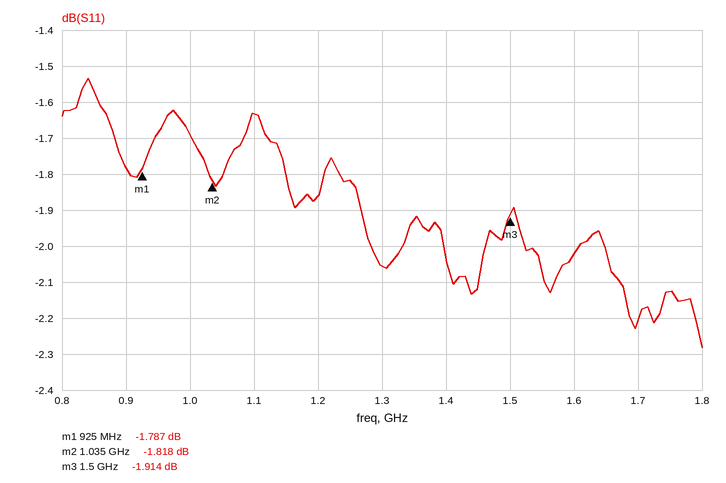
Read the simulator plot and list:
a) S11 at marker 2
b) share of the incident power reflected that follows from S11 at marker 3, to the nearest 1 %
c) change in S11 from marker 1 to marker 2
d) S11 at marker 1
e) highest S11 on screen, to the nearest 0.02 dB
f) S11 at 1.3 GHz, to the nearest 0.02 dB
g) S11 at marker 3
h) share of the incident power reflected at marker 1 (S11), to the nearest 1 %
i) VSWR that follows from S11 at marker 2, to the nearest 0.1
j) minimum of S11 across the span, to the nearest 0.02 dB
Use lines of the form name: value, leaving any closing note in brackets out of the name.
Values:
S11 at marker 2: -1.818 dB
share of the incident power reflected that follows from S11 at marker 3, to the nearest 1 %: 64 %
change in S11 from marker 1 to marker 2: -0.031 dB
S11 at marker 1: -1.787 dB
highest S11 on screen, to the nearest 0.02 dB: -1.54 dB
S11 at 1.3 GHz, to the nearest 0.02 dB: -2.06 dB
S11 at marker 3: -1.914 dB
share of the incident power reflected at marker 1 (S11), to the nearest 1 %: 66 %
VSWR that follows from S11 at marker 2, to the nearest 0.1: 9.6
minimum of S11 across the span, to the nearest 0.02 dB: -2.28 dB
